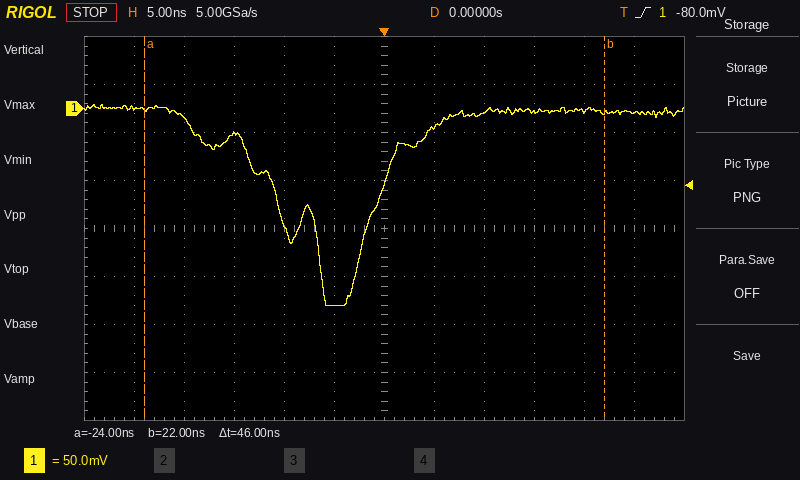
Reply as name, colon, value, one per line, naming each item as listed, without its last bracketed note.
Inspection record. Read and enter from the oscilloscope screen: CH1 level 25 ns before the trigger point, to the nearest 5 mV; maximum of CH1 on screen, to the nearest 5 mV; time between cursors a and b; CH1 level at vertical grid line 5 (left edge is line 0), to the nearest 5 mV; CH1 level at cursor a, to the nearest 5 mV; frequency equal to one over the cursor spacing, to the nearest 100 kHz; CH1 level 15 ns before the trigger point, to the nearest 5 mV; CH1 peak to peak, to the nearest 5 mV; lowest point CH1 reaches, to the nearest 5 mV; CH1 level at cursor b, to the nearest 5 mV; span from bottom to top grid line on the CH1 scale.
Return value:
CH1 level 25 ns before the trigger point, to the nearest 5 mV: 0 mV
maximum of CH1 on screen, to the nearest 5 mV: 5 mV
time between cursors a and b: 46 ns
CH1 level at vertical grid line 5 (left edge is line 0), to the nearest 5 mV: -205 mV
CH1 level at cursor a, to the nearest 5 mV: 0 mV
frequency equal to one over the cursor spacing, to the nearest 100 kHz: 21.7 MHz
CH1 level 15 ns before the trigger point, to the nearest 5 mV: -25 mV
CH1 peak to peak, to the nearest 5 mV: 210 mV
lowest point CH1 reaches, to the nearest 5 mV: -205 mV
CH1 level at cursor b, to the nearest 5 mV: -5 mV
span from bottom to top grid line on the CH1 scale: 400 mV
